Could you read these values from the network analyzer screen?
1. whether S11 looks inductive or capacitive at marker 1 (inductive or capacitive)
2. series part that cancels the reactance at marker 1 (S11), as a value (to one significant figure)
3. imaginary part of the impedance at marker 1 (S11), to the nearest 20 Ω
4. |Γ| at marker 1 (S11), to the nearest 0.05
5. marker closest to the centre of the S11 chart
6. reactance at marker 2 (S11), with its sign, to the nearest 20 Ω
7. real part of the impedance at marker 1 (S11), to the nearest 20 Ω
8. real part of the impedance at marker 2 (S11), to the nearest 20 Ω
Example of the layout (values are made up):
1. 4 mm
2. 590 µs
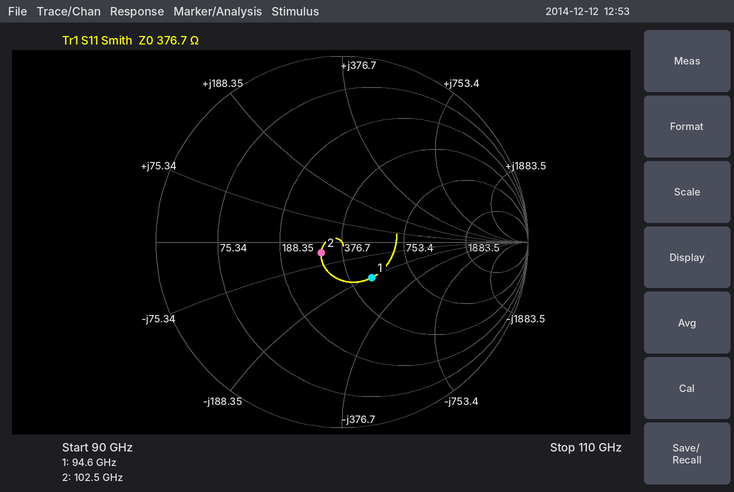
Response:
1. capacitive
2. 300 pH
3. -200 Ω
4. 0.25
5. marker 2
6. -40 Ω
7. 480 Ω
8. 300 Ω
